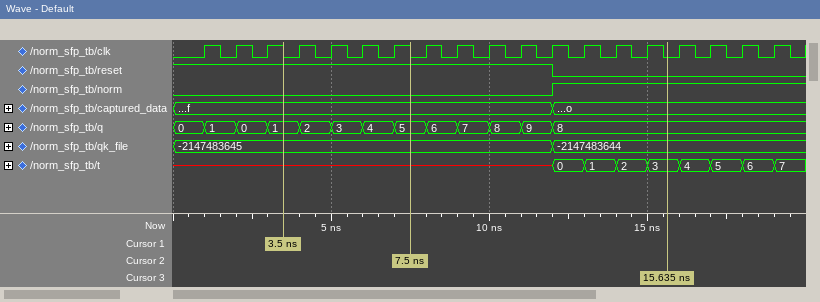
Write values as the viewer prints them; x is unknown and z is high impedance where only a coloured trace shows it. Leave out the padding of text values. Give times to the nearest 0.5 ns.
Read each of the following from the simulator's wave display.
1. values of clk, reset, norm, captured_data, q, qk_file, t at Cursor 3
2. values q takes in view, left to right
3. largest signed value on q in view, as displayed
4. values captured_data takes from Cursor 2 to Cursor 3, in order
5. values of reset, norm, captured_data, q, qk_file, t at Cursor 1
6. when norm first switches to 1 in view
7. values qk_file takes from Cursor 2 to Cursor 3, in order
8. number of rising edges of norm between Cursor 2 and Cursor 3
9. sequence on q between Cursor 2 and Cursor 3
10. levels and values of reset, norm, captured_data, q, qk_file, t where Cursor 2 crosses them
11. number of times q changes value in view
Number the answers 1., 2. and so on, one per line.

1. clk=0, reset=0, norm=1, captured_data=o, q=8, qk_file=-2147483644, t=3
2. 0, 1, 0, 1, 2, 3, 4, 5, 6, 7, 8, 9, 8
3. 9
4. f, o
5. reset=1, norm=0, captured_data=f, q=1, qk_file=-2147483645, t=x
6. 12 ns
7. -2147483645, -2147483644
8. 1
9. 5, 6, 7, 8, 9, 8
10. reset=1, norm=0, captured_data=f, q=5, qk_file=-2147483645, t=x
11. 12
